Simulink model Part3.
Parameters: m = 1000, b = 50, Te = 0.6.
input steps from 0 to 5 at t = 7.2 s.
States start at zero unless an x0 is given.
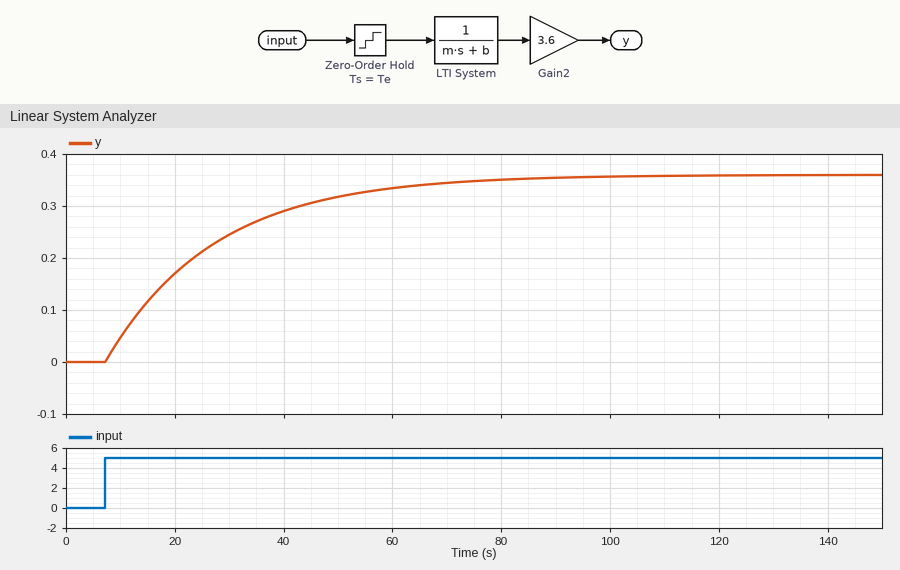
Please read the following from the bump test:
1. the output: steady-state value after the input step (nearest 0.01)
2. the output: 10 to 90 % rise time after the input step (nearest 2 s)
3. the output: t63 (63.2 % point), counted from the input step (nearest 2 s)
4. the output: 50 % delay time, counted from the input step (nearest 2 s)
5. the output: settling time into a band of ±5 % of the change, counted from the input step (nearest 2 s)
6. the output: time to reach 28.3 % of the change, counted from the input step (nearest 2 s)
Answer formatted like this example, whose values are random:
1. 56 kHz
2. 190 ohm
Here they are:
1. 0.36
2. 44 s
3. 20 s
4. 14 s
5. 60 s
6. 6 s
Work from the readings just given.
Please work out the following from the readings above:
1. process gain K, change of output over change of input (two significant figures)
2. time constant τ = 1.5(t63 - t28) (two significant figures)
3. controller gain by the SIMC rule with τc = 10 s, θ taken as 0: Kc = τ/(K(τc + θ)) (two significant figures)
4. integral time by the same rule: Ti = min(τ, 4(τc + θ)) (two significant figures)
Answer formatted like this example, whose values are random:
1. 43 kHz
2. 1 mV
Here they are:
1. 0.072
2. 21 s
3. 29
4. 21 s
